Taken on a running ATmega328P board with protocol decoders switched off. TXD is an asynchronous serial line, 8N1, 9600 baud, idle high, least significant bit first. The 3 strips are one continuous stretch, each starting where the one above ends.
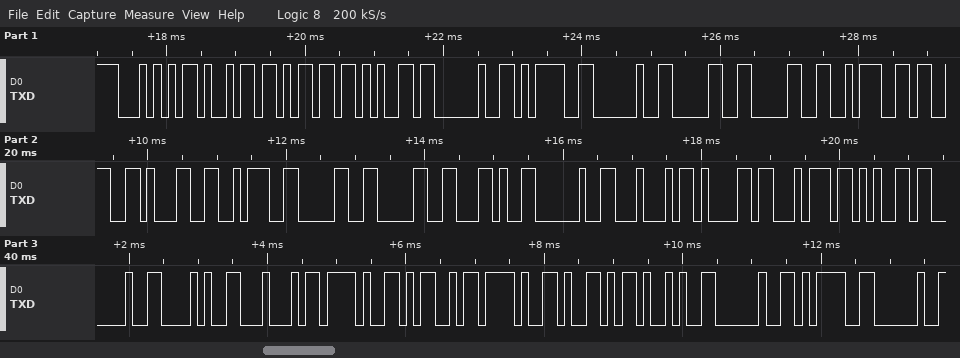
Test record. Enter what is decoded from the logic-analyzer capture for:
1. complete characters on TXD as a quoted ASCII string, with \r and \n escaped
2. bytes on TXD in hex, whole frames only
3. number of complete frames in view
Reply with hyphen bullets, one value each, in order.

- "Time = 00:31:00, Date (D/M/Y) = "
- 0x54 0x69 0x6D 0x65 0x20 0x3D 0x20 0x30 0x30 0x3A 0x33 0x31 0x3A 0x30 0x30 0x2C 0x20 0x44 0x61 0x74 0x65 0x20 0x28 0x44 0x2F 0x4D 0x2F 0x59 0x29 0x20 0x3D 0x20
- 32
